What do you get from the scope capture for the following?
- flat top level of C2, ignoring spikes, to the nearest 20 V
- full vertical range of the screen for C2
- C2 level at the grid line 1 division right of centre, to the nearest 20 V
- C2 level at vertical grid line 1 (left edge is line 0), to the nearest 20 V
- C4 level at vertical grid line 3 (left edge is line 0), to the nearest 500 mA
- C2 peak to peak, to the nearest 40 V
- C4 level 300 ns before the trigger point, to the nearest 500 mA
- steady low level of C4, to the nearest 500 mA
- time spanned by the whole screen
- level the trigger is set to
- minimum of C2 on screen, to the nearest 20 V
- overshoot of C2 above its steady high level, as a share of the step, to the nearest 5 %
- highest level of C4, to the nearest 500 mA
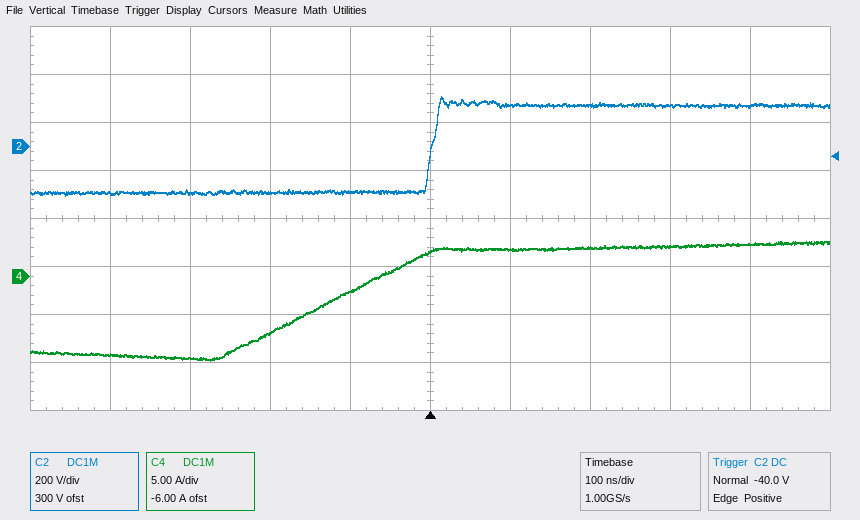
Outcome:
180 V
1.6 kV
180 V
-200 V
-6.0 A
400 V
-8.5 A
-8.5 A
1 µs
-40.0 V
-200 V
10 %
3.5 A
